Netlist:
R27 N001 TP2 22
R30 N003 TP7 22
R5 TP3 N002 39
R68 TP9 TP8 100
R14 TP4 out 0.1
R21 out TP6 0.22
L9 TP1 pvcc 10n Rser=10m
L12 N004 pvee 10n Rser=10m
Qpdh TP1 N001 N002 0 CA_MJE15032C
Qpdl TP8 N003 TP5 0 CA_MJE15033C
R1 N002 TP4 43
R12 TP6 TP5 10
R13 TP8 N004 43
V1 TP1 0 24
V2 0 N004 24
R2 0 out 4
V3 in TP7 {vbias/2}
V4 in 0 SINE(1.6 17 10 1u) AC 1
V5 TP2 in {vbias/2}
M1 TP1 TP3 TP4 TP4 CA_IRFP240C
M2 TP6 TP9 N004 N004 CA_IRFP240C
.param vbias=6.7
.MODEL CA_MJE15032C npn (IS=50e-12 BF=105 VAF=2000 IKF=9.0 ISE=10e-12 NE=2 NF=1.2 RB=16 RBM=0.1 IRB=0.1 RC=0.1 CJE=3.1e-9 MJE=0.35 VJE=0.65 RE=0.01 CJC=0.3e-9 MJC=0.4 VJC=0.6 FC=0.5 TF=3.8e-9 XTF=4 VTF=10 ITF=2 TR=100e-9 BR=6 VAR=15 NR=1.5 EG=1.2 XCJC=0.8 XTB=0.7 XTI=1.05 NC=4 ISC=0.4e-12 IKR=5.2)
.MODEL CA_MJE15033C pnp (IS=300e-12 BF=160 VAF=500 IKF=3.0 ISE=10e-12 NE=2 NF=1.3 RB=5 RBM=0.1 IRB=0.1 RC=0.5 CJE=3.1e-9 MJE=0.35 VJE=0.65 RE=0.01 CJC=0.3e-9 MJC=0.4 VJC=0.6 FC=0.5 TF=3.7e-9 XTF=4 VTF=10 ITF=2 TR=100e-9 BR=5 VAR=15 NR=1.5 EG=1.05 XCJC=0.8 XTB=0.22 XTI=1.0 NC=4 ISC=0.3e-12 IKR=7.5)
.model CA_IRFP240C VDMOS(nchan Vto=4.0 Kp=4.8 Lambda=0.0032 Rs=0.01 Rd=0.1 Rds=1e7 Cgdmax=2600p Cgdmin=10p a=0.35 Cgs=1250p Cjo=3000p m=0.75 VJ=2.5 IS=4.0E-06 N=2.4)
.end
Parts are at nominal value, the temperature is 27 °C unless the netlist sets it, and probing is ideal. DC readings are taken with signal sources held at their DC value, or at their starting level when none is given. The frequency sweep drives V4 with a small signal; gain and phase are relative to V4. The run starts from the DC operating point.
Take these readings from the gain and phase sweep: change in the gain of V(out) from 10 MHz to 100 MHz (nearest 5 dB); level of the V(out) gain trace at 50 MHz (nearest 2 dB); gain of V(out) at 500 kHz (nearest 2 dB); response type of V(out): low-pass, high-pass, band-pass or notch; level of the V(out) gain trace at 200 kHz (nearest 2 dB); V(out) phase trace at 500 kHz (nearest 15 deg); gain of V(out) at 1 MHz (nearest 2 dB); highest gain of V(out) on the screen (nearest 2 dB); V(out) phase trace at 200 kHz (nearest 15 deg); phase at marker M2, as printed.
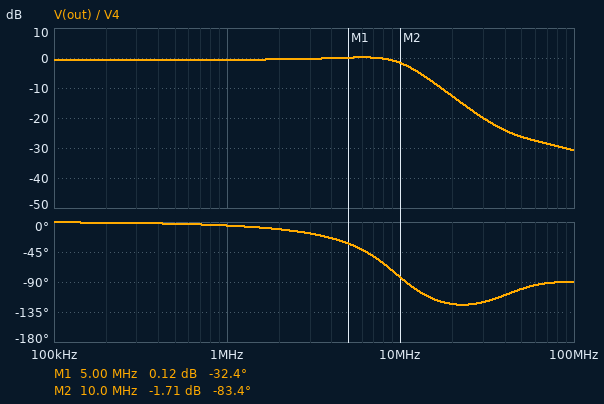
-30 dB
-26 dB
0 dB
low-pass
0 dB
0 deg
0 dB
0 dB
0 deg
-83.4 deg
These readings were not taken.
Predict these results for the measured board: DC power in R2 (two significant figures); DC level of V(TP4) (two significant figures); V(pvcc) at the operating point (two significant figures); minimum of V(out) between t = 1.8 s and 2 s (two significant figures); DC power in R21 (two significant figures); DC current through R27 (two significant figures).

96 µW
6.1 mV
24 V
-16 V
15 mW
980 µA
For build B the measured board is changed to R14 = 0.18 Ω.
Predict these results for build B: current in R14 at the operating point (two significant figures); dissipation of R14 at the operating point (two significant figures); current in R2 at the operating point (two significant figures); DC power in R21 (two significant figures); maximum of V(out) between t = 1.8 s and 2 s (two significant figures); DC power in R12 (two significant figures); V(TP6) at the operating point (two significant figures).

240 mA
11 mW
6.3 mA
14 mW
15 V
98 mW
-80 mV
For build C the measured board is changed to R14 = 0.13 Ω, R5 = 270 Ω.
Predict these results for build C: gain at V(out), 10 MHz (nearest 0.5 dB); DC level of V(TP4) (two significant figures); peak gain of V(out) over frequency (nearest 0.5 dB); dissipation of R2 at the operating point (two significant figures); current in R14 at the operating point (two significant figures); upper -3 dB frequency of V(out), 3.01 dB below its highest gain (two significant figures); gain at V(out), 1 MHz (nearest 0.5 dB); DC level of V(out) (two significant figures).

-6.5 dB
11 mV
0 dB
120 µW
250 mA
8.0 MHz
-1.0 dB
-22 mV
